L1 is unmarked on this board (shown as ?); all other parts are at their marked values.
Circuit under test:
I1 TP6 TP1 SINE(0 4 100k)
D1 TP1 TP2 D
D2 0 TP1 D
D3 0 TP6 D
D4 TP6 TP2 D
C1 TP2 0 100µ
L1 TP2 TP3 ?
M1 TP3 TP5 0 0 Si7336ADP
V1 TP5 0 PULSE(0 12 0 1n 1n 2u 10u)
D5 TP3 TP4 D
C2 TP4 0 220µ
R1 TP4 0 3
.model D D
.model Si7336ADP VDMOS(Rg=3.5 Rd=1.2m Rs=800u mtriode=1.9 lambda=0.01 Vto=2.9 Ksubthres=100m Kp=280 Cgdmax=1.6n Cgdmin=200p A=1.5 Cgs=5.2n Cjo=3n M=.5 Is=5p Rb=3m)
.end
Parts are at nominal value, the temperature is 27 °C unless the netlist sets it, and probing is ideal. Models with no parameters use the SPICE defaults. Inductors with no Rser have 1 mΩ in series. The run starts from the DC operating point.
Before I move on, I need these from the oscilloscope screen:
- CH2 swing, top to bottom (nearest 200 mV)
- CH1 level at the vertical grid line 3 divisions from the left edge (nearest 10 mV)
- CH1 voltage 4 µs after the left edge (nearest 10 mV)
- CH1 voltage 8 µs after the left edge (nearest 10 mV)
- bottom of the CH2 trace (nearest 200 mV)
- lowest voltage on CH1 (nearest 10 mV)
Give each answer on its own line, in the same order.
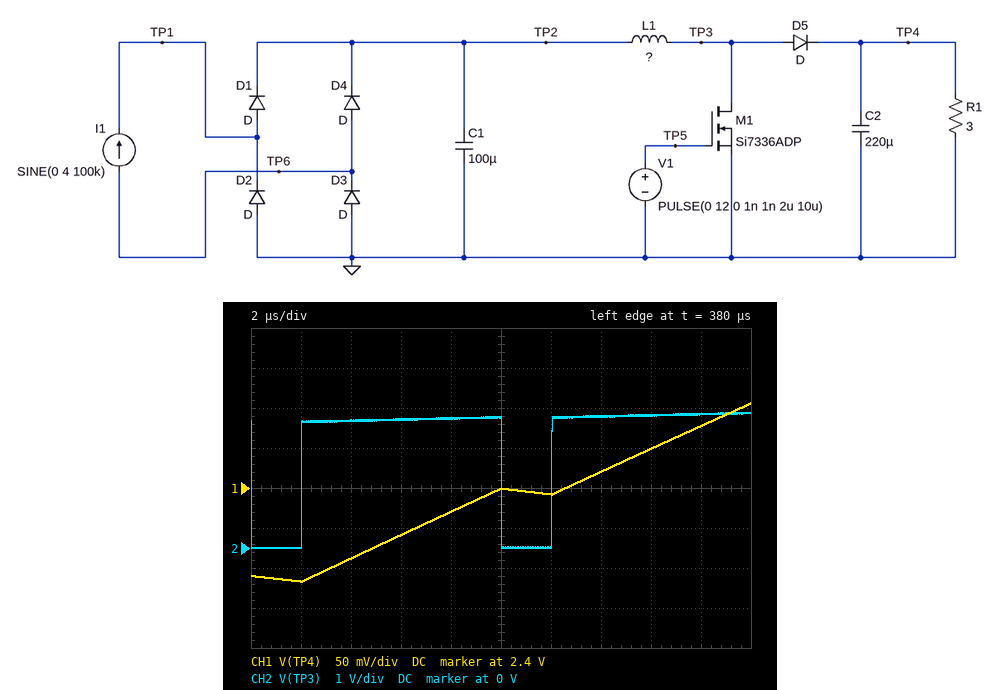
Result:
3.4 V
2.34 V
2.31 V
2.37 V
0 V
2.28 V
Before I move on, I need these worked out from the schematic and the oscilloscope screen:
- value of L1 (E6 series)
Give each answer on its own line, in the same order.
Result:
150 µH
